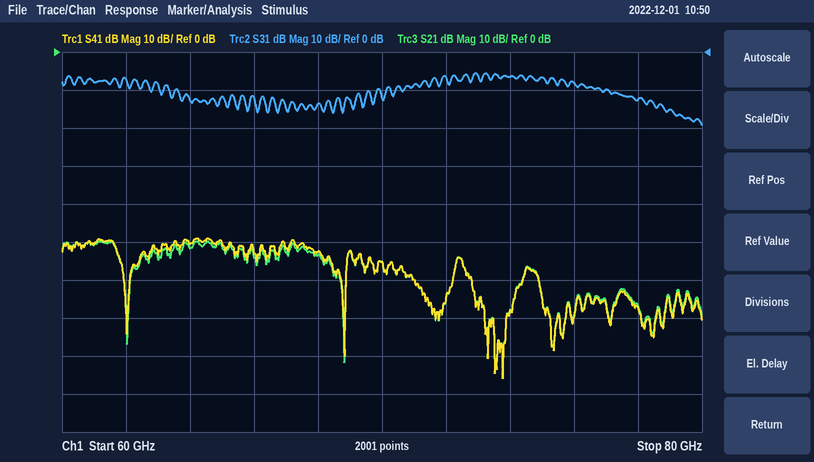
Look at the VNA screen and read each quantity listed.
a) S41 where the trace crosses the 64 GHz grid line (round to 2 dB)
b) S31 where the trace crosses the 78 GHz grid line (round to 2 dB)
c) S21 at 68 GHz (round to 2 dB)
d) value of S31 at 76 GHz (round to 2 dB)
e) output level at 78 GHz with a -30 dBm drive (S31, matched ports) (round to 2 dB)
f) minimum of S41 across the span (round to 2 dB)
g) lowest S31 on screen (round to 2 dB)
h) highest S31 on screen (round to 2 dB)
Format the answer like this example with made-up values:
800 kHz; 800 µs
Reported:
-50 dB; -12 dB; -54 dB; -8 dB; -42 dBm; -86 dB; -20 dB; -6 dB
